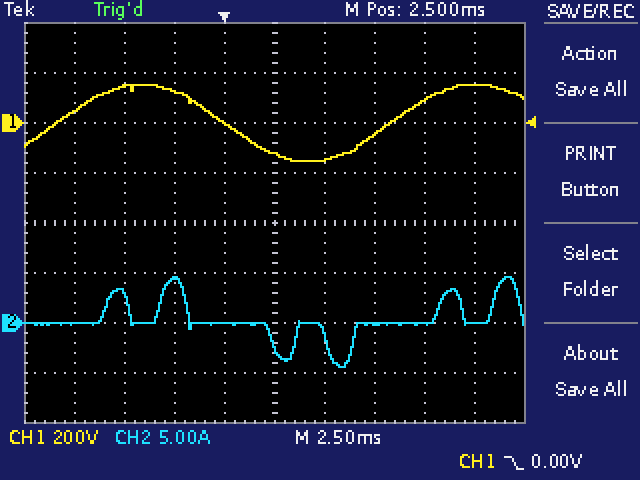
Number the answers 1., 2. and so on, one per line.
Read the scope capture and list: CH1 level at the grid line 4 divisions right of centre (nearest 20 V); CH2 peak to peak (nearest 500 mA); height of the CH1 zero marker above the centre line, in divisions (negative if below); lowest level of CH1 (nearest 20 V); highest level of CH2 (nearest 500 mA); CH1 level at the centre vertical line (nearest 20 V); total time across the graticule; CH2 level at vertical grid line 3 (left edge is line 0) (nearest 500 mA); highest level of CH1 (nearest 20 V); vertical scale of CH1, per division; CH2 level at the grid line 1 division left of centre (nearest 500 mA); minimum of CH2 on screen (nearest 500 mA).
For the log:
1. 160 V
2. 9.0 A
3. +2.0 div
4. -160 V
5. 4.5 A
6. -120 V
7. 25 ms
8. 4.5 A
9. 160 V
10. 200 V
11. 0.0 A
12. -4.5 A
